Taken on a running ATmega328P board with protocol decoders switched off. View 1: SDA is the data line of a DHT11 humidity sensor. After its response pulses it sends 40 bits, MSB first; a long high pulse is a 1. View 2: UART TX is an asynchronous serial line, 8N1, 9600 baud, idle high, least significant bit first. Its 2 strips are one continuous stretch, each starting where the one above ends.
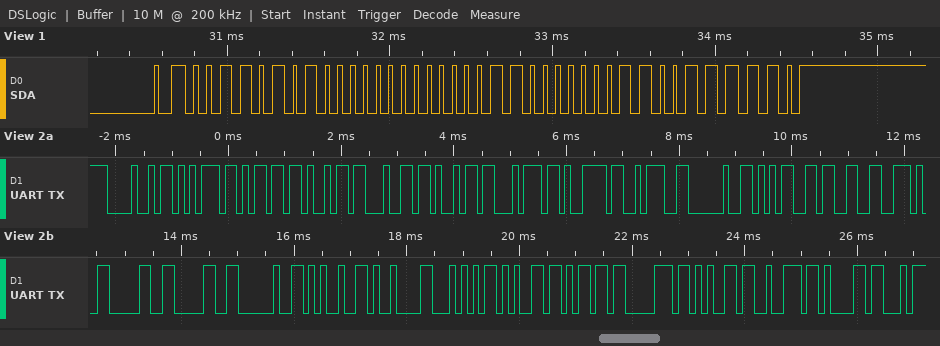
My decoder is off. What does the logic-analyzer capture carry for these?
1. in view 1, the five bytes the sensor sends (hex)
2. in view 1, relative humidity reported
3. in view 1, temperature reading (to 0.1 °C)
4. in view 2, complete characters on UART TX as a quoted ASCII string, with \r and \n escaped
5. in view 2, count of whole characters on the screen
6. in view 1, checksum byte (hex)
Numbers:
35 00 06 03 3E
53 %
6.3 °C
"Humidity: 53.00 %\tTempera"
25
0x3E
